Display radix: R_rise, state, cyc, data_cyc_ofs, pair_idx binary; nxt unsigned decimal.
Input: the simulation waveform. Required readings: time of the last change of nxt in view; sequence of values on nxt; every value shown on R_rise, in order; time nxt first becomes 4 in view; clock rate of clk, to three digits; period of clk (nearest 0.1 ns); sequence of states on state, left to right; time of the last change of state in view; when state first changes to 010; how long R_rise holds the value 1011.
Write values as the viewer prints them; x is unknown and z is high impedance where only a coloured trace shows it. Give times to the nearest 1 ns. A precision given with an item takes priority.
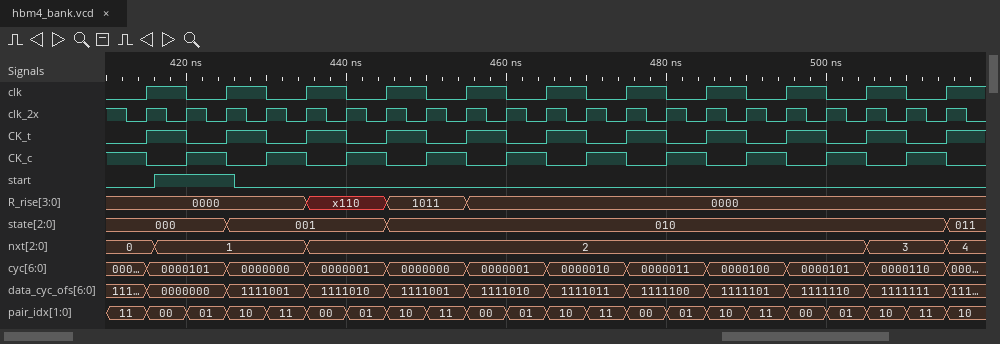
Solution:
515 ns
0, 1, 2, 3, 4
0000, x110, 1011, 0000
515 ns
100 MHz
10 ns
000, 001, 010, 011
515 ns
445 ns
10 ns
